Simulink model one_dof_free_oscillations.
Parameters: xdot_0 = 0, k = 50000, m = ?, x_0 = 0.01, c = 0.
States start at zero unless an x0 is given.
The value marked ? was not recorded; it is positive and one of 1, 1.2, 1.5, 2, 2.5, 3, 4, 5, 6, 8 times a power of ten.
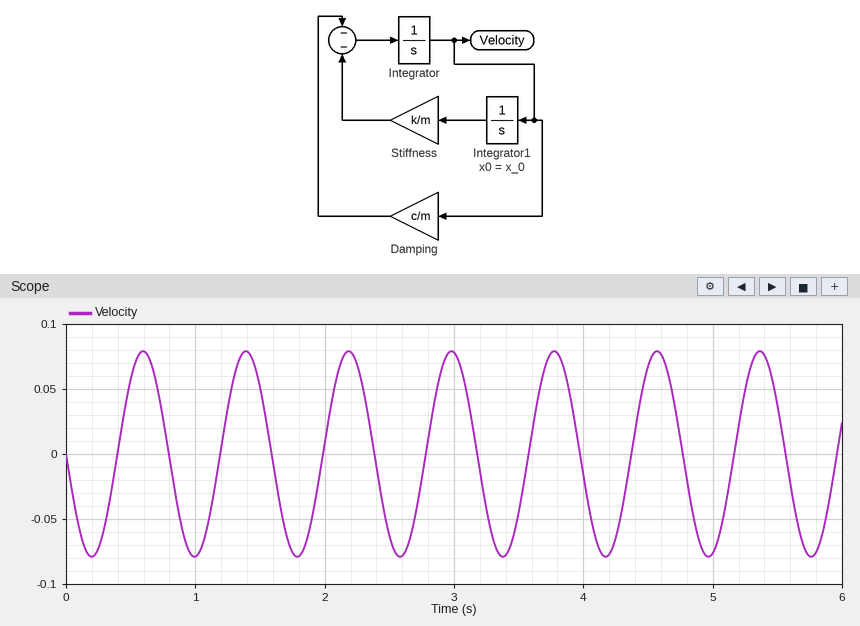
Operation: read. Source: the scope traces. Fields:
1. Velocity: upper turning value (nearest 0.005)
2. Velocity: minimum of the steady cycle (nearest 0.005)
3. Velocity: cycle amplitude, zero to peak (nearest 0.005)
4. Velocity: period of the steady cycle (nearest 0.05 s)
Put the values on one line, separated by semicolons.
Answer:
0.080; -0.080; 0.080; 0.80 s
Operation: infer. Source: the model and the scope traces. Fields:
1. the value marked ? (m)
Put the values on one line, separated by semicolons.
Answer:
800
